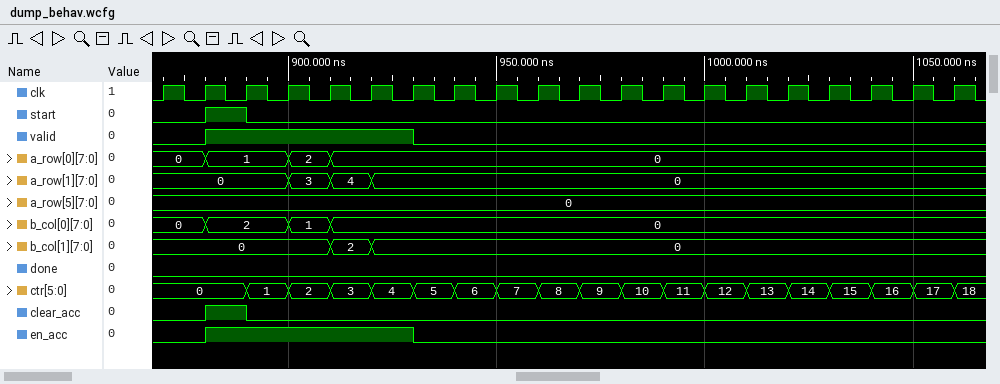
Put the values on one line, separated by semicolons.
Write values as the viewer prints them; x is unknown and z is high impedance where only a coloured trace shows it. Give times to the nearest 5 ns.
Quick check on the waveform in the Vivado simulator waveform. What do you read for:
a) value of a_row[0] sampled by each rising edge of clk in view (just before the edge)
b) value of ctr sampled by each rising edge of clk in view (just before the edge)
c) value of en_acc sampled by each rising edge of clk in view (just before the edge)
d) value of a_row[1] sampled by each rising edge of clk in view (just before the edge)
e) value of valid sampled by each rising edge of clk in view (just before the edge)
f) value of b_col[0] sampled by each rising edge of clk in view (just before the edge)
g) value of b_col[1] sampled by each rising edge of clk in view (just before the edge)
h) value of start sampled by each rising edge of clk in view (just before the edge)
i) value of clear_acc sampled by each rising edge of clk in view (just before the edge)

0, 0, 1, 1, 2, 0, 0, 0, 0, 0, 0, 0, 0, 0, 0, 0, 0, 0, 0, 0; 0, 0, 0, 1, 2, 3, 4, 5, 6, 7, 8, 9, 10, 11, 12, 13, 14, 15, 16, 17; 0 0 1 1 1 1 1 0 0 0 0 0 0 0 0 0 0 0 0 0; 0, 0, 0, 0, 3, 4, 0, 0, 0, 0, 0, 0, 0, 0, 0, 0, 0, 0, 0, 0; 0 0 1 1 1 1 1 0 0 0 0 0 0 0 0 0 0 0 0 0; 0, 0, 2, 2, 1, 0, 0, 0, 0, 0, 0, 0, 0, 0, 0, 0, 0, 0, 0, 0; 0, 0, 0, 0, 0, 2, 0, 0, 0, 0, 0, 0, 0, 0, 0, 0, 0, 0, 0, 0; 0 0 1 0 0 0 0 0 0 0 0 0 0 0 0 0 0 0 0 0; 0 0 1 0 0 0 0 0 0 0 0 0 0 0 0 0 0 0 0 0
